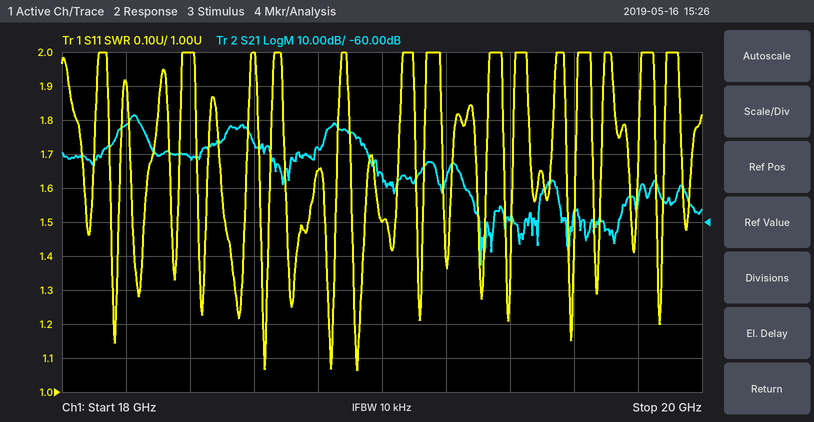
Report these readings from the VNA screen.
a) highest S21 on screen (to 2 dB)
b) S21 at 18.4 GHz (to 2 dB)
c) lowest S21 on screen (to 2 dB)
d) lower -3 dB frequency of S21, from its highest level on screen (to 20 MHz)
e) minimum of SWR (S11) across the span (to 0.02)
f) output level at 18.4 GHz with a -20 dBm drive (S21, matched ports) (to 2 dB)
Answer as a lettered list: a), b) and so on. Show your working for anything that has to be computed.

a) -28 dB
b) -40 dB
c) -72 dB
d) 18.20 GHz
e) 1.06
f) -20 dBm + (-40 dB) = -60 dBm
